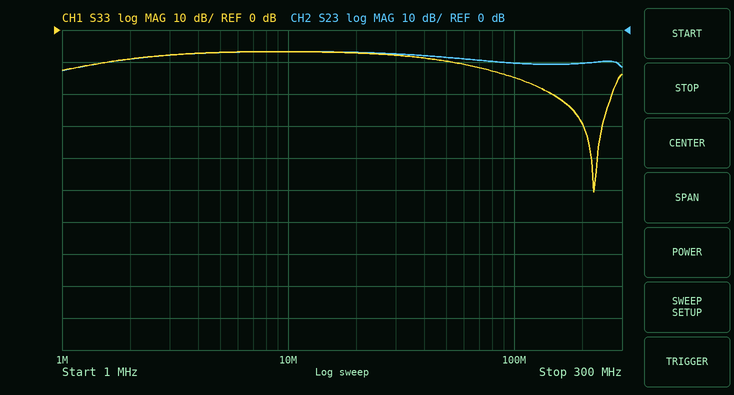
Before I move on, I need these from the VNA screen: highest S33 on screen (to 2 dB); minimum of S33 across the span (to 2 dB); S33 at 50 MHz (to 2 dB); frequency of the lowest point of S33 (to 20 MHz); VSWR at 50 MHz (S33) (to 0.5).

-6 dB
-50 dB
-10 dB
220 MHz
2.0
